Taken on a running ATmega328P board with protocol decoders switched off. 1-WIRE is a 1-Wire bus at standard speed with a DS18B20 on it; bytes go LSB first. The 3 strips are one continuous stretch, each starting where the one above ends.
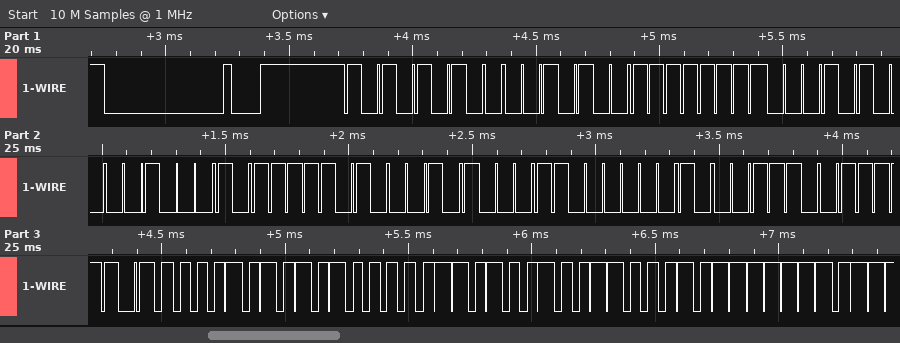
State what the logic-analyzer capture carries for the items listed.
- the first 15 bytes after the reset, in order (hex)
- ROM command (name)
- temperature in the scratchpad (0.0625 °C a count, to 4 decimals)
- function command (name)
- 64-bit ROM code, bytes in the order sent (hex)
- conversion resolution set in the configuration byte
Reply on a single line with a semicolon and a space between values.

55 28 FF 28 44 5F 14 03 71 BE 50 05 4B 46 7F; Match ROM; 85.0000 °C; Read Scratchpad; 28 FF 28 44 5F 14 03 71; 12 bits
